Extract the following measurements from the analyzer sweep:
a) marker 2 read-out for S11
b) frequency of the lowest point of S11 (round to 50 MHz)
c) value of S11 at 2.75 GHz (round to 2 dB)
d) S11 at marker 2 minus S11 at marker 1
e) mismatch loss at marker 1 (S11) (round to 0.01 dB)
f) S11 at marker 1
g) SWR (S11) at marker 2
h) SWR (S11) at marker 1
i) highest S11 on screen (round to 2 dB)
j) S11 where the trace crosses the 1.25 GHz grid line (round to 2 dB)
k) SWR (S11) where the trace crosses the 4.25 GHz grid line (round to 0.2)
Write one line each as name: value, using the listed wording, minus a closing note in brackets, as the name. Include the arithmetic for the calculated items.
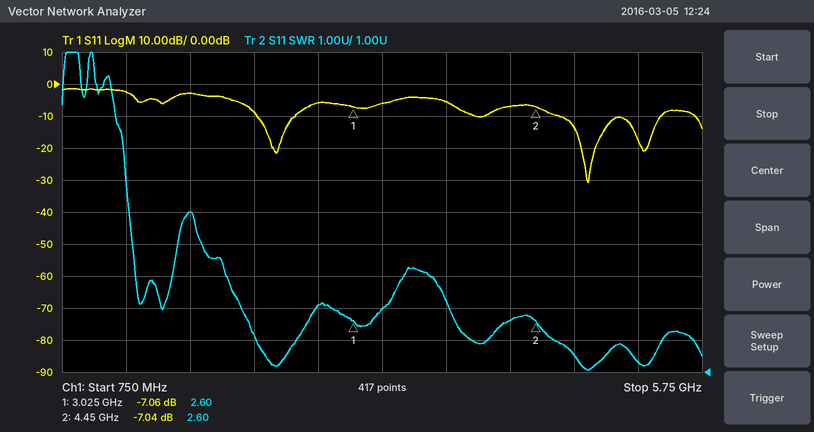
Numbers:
marker 2 read-out for S11: -7.04 dB
frequency of the lowest point of S11: 4.85 GHz
value of S11 at 2.75 GHz: -6 dB
S11 at marker 2 minus S11 at marker 1: -7.04 − (-7.06) = 0.02 dB
mismatch loss at marker 1 (S11): −10 log10(1 − 10^(-7.06/10)) ≈ 0.95 dB
S11 at marker 1: -7.06 dB
SWR (S11) at marker 2: 2.60
SWR (S11) at marker 1: 2.60
highest S11 on screen: -2 dB
S11 where the trace crosses the 1.25 GHz grid line: -2 dB
SWR (S11) where the trace crosses the 4.25 GHz grid line: 2.6
